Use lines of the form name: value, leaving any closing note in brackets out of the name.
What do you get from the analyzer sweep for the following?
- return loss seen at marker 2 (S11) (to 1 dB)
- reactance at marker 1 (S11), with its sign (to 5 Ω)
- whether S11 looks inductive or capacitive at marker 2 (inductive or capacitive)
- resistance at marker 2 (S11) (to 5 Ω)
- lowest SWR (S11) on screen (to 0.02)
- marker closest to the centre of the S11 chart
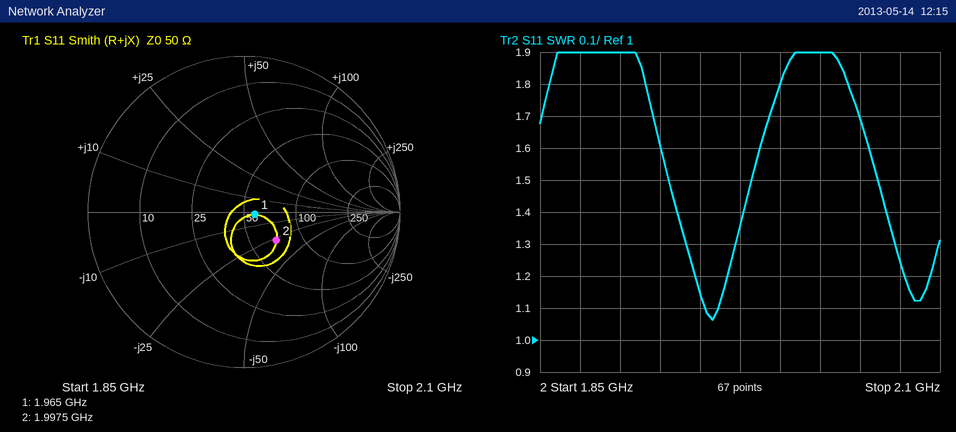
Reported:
return loss seen at marker 2 (S11): 11 dB
reactance at marker 1 (S11), with its sign: 0 Ω
whether S11 looks inductive or capacitive at marker 2: capacitive
resistance at marker 2 (S11): 70 Ω
lowest SWR (S11) on screen: 1.06
marker closest to the centre of the S11 chart: marker 1
